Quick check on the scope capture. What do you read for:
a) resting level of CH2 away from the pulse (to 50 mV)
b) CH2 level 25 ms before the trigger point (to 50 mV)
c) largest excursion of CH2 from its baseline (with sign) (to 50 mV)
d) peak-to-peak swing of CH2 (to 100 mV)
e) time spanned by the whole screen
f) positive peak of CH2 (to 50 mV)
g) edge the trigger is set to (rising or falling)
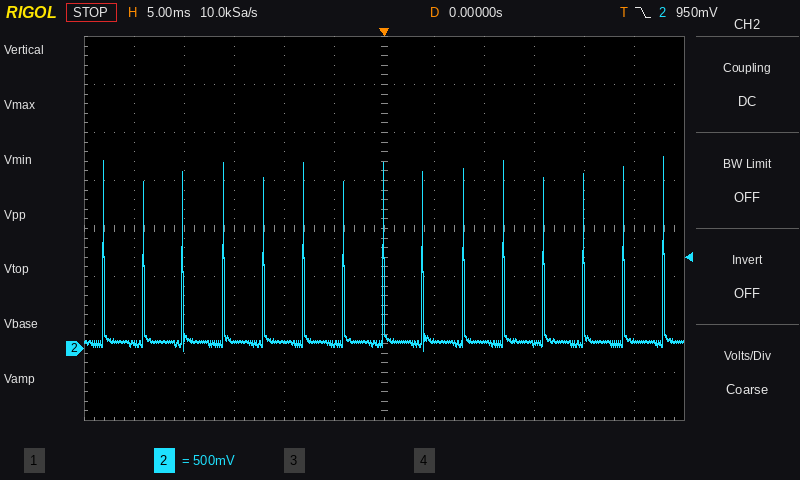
50 mV
50 mV
+1.95 V
2.00 V
60 ms
2.00 V
falling
